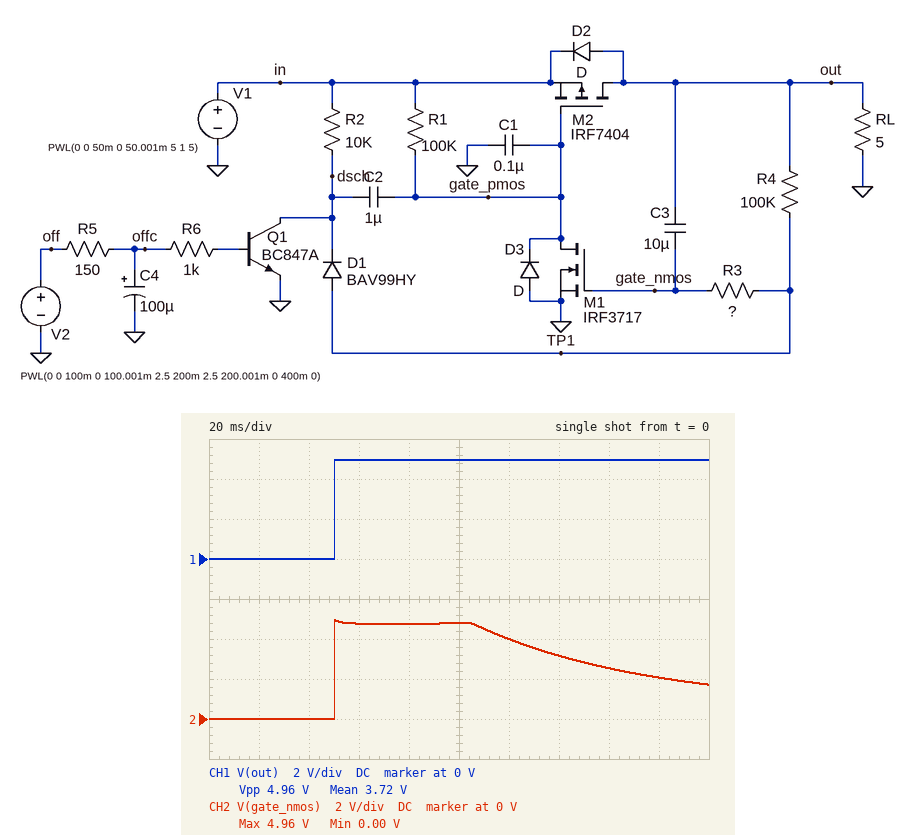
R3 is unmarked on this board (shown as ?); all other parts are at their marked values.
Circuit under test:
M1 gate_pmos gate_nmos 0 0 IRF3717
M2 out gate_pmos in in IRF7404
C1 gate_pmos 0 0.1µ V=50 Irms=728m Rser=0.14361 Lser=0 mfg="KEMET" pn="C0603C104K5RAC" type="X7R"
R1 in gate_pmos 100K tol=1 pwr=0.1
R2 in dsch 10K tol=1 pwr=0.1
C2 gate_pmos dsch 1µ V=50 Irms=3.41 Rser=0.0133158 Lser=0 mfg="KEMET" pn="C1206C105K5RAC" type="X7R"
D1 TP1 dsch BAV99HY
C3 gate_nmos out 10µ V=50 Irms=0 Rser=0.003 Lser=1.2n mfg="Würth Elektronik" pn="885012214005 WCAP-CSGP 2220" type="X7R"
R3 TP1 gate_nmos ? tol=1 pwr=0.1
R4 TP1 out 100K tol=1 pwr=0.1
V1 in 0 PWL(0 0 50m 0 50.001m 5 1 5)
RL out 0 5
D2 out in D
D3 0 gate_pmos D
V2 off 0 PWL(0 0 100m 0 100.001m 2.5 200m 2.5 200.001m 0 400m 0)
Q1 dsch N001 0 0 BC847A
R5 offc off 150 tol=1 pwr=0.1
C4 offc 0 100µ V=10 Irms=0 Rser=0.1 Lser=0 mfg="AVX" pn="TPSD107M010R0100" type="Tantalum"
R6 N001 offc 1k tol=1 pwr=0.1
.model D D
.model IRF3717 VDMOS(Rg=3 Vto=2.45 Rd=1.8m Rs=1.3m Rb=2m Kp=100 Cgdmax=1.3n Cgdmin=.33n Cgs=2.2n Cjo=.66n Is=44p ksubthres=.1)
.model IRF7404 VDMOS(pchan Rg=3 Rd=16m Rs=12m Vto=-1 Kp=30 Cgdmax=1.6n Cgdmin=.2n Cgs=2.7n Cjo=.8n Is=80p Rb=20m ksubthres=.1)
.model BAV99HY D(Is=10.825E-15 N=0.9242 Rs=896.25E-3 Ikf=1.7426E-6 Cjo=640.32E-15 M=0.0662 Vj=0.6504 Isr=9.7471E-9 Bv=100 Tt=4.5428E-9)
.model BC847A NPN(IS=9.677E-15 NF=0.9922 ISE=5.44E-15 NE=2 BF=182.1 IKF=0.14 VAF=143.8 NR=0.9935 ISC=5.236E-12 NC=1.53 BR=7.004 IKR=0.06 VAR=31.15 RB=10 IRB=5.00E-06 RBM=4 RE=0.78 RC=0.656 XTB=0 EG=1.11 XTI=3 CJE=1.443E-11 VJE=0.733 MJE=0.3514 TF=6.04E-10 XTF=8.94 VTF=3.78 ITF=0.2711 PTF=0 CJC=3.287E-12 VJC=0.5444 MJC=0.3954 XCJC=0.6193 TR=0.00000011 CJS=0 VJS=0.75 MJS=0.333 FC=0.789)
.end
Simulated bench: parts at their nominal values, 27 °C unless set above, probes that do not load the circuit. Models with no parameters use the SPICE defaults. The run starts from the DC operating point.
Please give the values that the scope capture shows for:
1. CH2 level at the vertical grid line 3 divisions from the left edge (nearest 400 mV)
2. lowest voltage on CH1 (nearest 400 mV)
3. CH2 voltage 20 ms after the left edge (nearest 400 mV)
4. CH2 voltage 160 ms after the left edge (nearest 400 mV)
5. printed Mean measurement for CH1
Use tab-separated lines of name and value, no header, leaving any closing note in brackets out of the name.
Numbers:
CH2 level at the vertical grid line 3 divisions from the left edge	4.8 V
lowest voltage on CH1	0 V
CH2 voltage 20 ms after the left edge	0 V
CH2 voltage 160 ms after the left edge	2.4 V
printed Mean measurement for CH1	3.72 V
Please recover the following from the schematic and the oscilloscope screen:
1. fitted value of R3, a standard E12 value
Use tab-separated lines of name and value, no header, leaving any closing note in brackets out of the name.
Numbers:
fitted value of R3, a standard E12 value	6.8 kΩ
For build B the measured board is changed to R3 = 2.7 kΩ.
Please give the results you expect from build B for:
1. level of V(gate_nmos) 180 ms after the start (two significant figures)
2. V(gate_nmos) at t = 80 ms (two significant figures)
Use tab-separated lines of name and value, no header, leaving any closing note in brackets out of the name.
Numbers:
level of V(gate_nmos) 180 ms after the start	950 mV
V(gate_nmos) at t = 80 ms	4.7 V
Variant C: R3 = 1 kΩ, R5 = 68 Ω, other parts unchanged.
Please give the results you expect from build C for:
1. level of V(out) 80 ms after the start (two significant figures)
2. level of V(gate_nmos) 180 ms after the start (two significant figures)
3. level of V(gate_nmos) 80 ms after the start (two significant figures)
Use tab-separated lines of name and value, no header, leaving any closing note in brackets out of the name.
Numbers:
level of V(out) 80 ms after the start	5.0 V
level of V(gate_nmos) 180 ms after the start	620 mV
level of V(gate_nmos) 80 ms after the start	4.6 V
